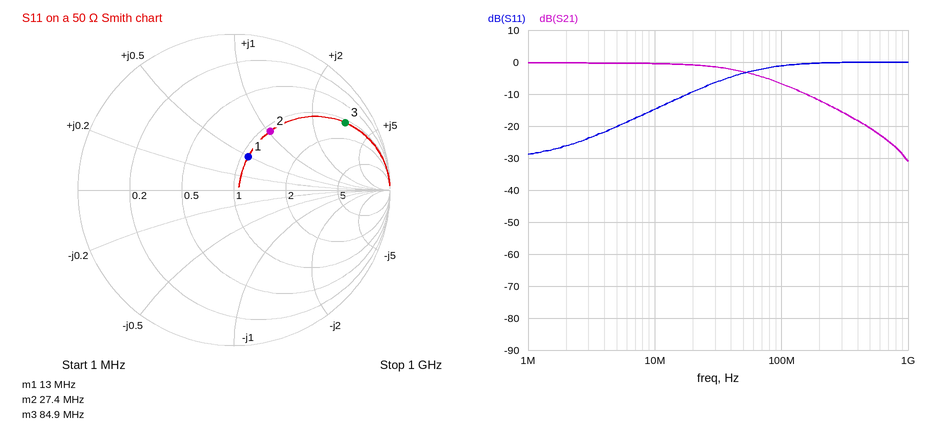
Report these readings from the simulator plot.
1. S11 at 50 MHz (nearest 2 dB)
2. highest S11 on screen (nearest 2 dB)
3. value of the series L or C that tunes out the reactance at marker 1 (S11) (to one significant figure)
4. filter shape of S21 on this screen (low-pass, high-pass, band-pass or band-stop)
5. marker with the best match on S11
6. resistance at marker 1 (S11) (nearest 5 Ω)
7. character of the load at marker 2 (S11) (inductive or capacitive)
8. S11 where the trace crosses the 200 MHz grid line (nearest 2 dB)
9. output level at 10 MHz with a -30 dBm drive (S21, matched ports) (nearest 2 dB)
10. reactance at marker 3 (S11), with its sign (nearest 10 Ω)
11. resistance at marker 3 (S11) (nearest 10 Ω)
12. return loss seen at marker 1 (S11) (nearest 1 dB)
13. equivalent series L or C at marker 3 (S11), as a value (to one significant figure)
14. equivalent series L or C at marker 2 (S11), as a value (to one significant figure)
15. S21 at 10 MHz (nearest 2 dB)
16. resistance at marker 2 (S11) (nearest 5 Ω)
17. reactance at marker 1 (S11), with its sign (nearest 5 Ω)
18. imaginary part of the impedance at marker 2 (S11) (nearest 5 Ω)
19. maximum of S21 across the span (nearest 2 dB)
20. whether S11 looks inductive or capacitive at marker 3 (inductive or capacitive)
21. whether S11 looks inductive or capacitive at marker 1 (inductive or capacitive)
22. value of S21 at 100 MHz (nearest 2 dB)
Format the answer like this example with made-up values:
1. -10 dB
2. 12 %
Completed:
1. -4 dB
2. 0 dB
3. 500 pF
4. low-pass
5. marker 1
6. 55 Ω
7. inductive
8. 0 dB
9. -30 dBm
10. +160 Ω
11. 60 Ω
12. 13 dB
13. 300 nH
14. 300 nH
15. 0 dB
16. 55 Ω
17. +25 Ω
18. +50 Ω
19. 0 dB
20. inductive
21. inductive
22. -6 dB
